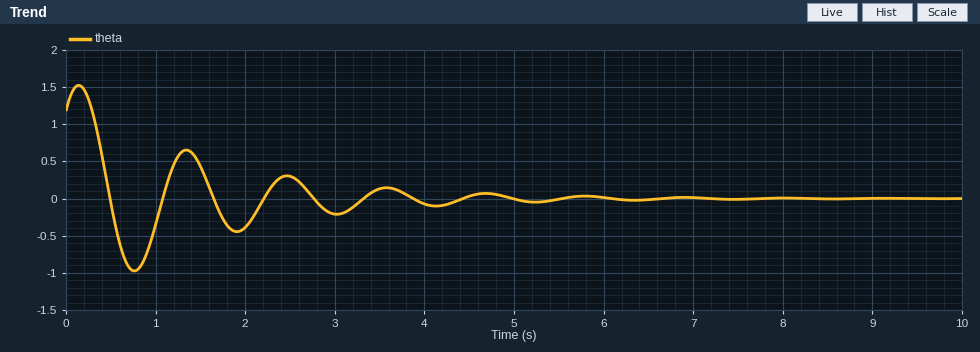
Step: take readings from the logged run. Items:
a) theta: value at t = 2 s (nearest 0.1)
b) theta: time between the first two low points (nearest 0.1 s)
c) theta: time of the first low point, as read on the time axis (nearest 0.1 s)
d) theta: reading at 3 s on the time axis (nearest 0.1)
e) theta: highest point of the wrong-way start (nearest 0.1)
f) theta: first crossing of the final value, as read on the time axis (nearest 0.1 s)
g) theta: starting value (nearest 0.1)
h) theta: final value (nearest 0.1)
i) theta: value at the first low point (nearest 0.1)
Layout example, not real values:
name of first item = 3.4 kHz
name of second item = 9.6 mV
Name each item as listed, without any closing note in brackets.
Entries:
theta: value at t = 2 s = -0.4
theta: time between the first two low points = 1.1 s
theta: time of the first low point, as read on the time axis = 0.8 s
theta: reading at 3 s on the time axis = -0.2
theta: highest point of the wrong-way start = 1.5
theta: first crossing of the final value, as read on the time axis = 0.5 s
theta: starting value = 1.2
theta: final value = 0.0
theta: value at the first low point = -1.0
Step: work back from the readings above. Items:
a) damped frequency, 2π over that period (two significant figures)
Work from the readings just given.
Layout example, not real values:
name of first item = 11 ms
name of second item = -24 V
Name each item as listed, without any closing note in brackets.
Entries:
damped frequency, 2π over that period = 5.7 rad/s
